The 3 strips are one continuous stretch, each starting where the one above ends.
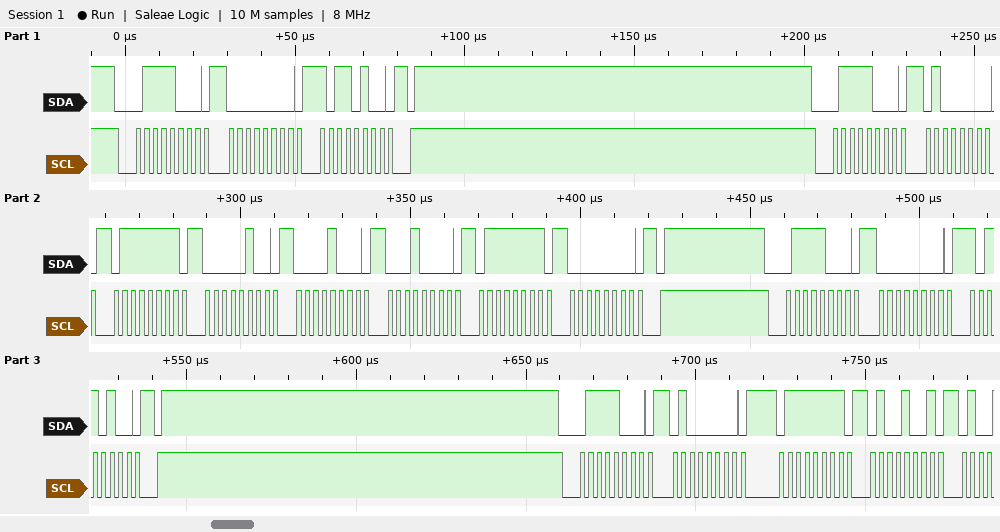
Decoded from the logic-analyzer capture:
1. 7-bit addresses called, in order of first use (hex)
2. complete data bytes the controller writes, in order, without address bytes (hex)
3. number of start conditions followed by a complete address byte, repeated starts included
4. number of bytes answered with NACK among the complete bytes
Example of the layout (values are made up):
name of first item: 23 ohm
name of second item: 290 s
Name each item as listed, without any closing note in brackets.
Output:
7-bit addresses called, in order of first use: 0x3C
complete data bytes the controller writes, in order, without address bytes: 00 B4 40 7F 04 08 10 7F 00 00 B4 40 7F 49
number of start conditions followed by a complete address byte, repeated starts included: 4
number of bytes answered with NACK among the complete bytes: 0
